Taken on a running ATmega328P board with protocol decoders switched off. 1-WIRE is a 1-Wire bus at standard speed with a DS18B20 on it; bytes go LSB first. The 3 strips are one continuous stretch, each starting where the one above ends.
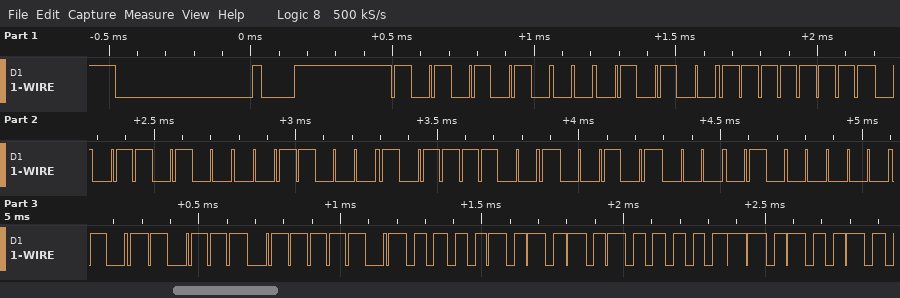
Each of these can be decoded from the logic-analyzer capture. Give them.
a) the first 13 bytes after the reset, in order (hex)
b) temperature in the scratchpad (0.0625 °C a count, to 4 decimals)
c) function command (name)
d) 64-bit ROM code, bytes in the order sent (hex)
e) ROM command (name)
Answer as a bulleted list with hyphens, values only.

- 55 28 FF 2C 8C 9E 14 02 ED BE 50 05 4B
- 85.0000 °C
- Read Scratchpad
- 28 FF 2C 8C 9E 14 02 ED
- Match ROM
